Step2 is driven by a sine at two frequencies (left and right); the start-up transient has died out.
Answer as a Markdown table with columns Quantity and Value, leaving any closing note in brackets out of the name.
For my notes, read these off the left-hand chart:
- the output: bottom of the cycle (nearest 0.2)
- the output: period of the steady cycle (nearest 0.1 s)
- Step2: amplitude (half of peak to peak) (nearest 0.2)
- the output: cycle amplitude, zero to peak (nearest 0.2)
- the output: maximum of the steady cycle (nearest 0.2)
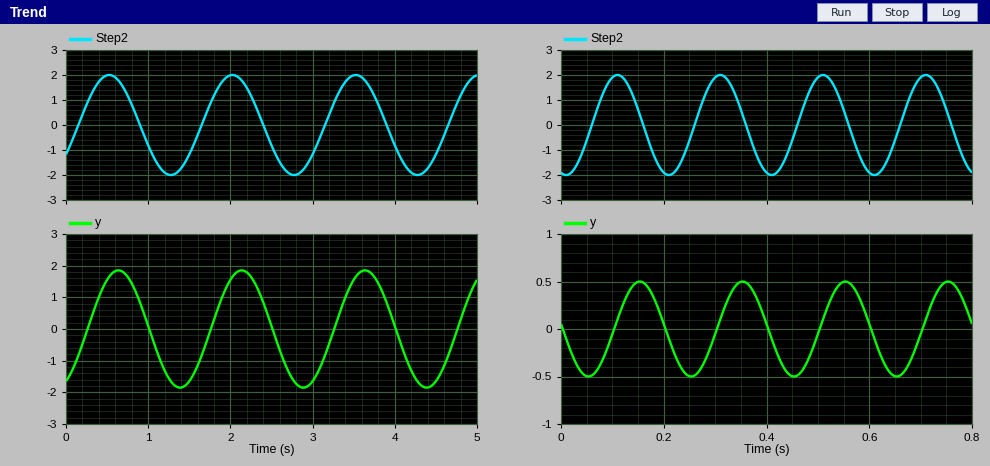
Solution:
| Quantity | Value |
|---|---|
| the output: bottom of the cycle | -1.8 |
| the output: period of the steady cycle | 1.5 s |
| Step2: amplitude (half of peak to peak) | 2.0 |
| the output: cycle amplitude, zero to peak | 1.8 |
| the output: maximum of the steady cycle | 1.8 |
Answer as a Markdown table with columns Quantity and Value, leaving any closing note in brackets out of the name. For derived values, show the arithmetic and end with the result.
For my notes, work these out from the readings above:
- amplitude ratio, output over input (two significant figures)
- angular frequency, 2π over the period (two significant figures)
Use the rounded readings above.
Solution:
| Quantity | Value |
|---|---|
| amplitude ratio, output over input | 1.8 / 2 = 0.90 |
| angular frequency, 2π over the period | 2π / 1.5 = 4.2 rad/s |
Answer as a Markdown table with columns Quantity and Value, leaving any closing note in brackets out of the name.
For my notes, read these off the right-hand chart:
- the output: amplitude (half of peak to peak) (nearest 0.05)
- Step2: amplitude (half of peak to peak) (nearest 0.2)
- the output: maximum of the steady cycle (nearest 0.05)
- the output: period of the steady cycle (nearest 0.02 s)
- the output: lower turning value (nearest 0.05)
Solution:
| Quantity | Value |
|---|---|
| the output: amplitude (half of peak to peak) | 0.50 |
| Step2: amplitude (half of peak to peak) | 2.0 |
| the output: maximum of the steady cycle | 0.50 |
| the output: period of the steady cycle | 0.20 s |
| the output: lower turning value | -0.50 |
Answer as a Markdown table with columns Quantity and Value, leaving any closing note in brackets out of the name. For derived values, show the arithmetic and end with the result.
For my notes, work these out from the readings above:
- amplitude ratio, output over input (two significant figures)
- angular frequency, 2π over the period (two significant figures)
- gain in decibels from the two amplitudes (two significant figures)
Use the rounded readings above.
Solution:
| Quantity | Value |
|---|---|
| amplitude ratio, output over input | 0.5 / 2 = 0.25 |
| angular frequency, 2π over the period | 2π / 0.2 = 31 rad/s |
| gain in decibels from the two amplitudes | 20 log10(0.5 / 2) = -12 dB |
